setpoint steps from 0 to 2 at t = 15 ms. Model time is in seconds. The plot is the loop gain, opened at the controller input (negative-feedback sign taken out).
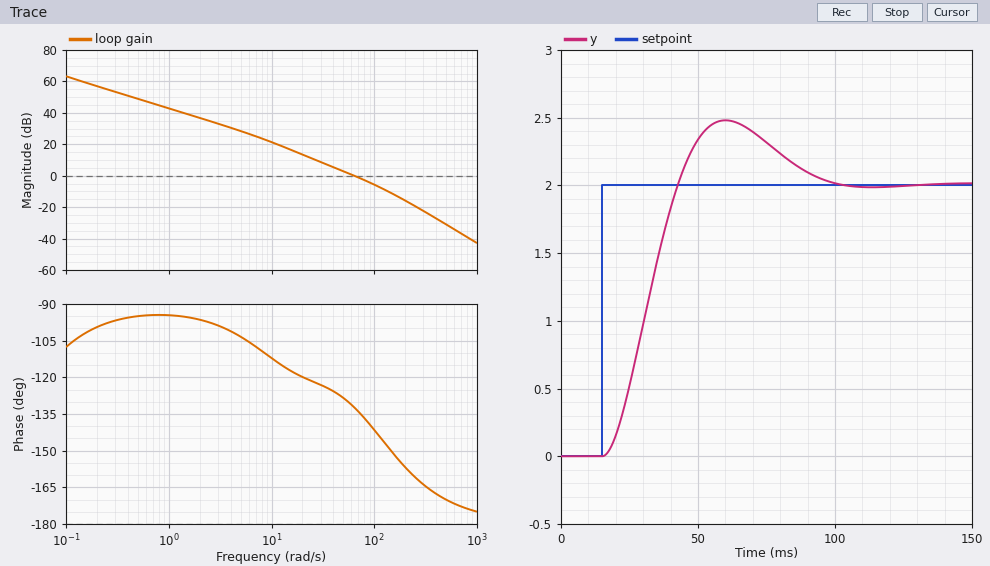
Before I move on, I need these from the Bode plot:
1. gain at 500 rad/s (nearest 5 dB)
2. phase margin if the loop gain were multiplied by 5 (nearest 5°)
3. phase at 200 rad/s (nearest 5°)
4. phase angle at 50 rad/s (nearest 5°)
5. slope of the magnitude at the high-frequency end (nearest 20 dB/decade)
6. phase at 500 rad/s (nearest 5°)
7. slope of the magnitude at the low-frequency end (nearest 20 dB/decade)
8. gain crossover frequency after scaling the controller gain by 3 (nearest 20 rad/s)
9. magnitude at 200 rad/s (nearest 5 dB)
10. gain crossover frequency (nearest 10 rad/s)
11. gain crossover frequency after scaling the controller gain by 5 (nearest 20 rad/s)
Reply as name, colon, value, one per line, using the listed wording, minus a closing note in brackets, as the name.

gain at 500 rad/s: -30 dB
phase margin if the loop gain were multiplied by 5: 25°
phase at 200 rad/s: -155°
phase angle at 50 rad/s: -130°
slope of the magnitude at the high-frequency end: -40 dB/decade
phase at 500 rad/s: -170°
slope of the magnitude at the low-frequency end: -20 dB/decade
gain crossover frequency after scaling the controller gain by 3: 140 rad/s
magnitude at 200 rad/s: -15 dB
gain crossover frequency: 60 rad/s
gain crossover frequency after scaling the controller gain by 5: 180 rad/s
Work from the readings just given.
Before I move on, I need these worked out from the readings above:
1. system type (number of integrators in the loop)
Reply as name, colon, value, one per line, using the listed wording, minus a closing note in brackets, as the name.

system type: 1
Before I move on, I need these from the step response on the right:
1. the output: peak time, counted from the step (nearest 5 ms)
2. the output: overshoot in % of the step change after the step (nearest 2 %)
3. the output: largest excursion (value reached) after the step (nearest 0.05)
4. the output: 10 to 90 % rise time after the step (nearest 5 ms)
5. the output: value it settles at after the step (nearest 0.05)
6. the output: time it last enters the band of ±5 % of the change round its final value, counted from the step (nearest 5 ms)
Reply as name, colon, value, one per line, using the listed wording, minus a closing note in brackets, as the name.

the output: peak time, counted from the step: 45 ms
the output: overshoot in % of the step change after the step: 24 %
the output: largest excursion (value reached) after the step: 2.50
the output: 10 to 90 % rise time after the step: 20 ms
the output: value it settles at after the step: 2.00
the output: time it last enters the band of ±5 % of the change round its final value, counted from the step: 75 ms
